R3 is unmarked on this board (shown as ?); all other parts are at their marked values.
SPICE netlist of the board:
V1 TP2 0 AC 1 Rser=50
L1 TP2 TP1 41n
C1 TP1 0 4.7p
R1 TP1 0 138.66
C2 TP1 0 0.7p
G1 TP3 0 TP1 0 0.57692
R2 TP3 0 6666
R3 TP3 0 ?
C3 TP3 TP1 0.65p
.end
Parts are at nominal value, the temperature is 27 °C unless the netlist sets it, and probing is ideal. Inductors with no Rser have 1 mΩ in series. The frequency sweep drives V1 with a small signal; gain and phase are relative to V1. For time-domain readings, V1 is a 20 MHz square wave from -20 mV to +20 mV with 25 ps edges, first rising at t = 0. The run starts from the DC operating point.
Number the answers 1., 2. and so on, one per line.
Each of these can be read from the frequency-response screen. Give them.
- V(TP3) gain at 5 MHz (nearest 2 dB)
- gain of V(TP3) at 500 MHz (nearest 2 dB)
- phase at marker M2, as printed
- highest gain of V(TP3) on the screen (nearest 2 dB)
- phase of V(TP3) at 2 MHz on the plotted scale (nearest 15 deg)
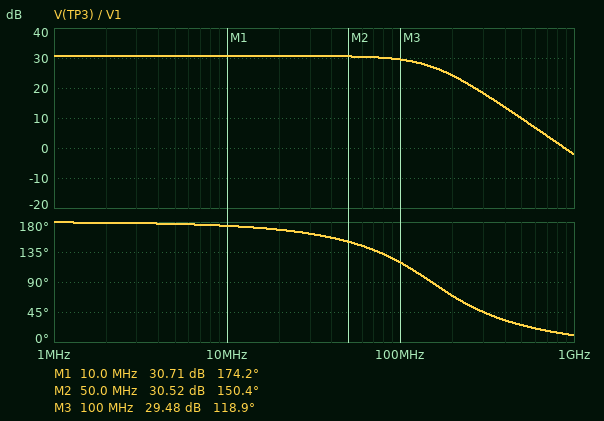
1. 30 dB
2. 10 dB
3. 150.4 deg
4. 30 dB
5. 180 deg
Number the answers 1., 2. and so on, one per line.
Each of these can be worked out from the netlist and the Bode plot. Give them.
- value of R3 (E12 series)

1. 82 Ω
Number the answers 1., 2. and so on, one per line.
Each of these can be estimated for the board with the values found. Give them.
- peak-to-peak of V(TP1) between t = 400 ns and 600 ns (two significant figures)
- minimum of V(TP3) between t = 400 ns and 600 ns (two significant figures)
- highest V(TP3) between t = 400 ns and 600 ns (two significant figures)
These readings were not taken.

1. 31 mV
2. -720 mV
3. 720 mV
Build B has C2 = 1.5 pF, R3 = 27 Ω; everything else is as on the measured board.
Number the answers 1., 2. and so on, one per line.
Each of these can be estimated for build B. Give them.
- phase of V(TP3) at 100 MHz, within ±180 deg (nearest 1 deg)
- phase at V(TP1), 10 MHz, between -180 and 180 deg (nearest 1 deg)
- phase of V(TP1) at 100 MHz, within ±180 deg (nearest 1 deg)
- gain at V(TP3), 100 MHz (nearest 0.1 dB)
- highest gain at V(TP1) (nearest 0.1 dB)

1. 146 deg
2. -3 deg
3. -33 deg
4. 21.5 dB
5. -2.3 dB
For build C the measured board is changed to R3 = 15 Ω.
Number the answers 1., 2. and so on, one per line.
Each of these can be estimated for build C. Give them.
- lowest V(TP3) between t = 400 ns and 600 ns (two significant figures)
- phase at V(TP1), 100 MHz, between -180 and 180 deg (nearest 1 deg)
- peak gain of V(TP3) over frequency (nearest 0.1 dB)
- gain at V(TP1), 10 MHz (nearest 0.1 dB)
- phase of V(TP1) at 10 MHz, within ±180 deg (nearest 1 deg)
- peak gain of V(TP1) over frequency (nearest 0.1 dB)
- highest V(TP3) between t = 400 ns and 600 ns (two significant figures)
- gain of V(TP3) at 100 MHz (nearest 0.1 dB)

1. -160 mV
2. -25 deg
3. 16.8 dB
4. -2.7 dB
5. -2 deg
6. -1.9 dB
7. 160 mV
8. 16.5 dB
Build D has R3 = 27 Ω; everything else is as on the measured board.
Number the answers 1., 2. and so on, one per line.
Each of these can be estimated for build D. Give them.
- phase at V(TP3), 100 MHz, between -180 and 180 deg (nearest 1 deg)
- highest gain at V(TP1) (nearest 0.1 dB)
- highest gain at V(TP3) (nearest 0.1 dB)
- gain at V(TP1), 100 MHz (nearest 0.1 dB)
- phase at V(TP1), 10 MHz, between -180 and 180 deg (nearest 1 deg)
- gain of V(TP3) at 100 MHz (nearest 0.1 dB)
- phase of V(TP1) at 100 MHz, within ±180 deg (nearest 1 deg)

1. 147 deg
2. -2.2 dB
3. 21.6 dB
4. -2.3 dB
5. -3 deg
6. 21.5 dB
7. -32 deg
